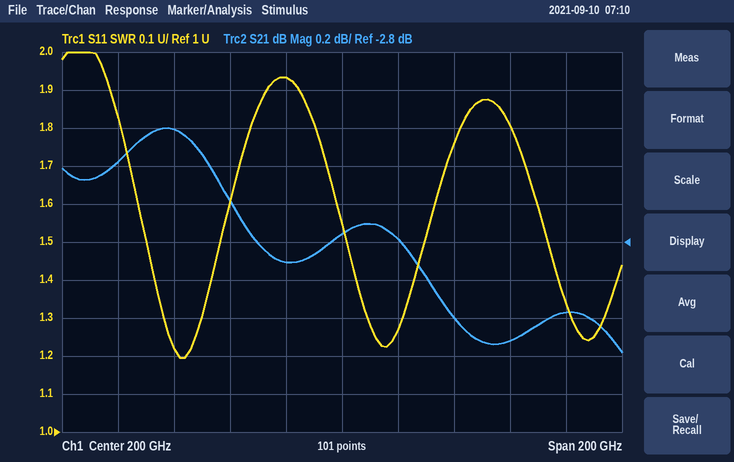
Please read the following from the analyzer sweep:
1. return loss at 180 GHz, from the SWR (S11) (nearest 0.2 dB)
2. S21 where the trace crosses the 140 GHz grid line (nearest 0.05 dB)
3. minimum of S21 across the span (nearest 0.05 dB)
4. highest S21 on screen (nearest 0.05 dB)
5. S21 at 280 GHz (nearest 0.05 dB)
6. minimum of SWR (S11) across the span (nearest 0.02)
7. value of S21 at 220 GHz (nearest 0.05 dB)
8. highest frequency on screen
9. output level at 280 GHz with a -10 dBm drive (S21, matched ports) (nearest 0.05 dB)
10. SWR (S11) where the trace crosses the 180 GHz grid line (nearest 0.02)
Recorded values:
10.0 dB
-2.20 dB
-3.40 dB
-2.20 dB
-3.15 dB
1.20
-2.80 dB
300 GHz
-13.15 dBm
1.94
